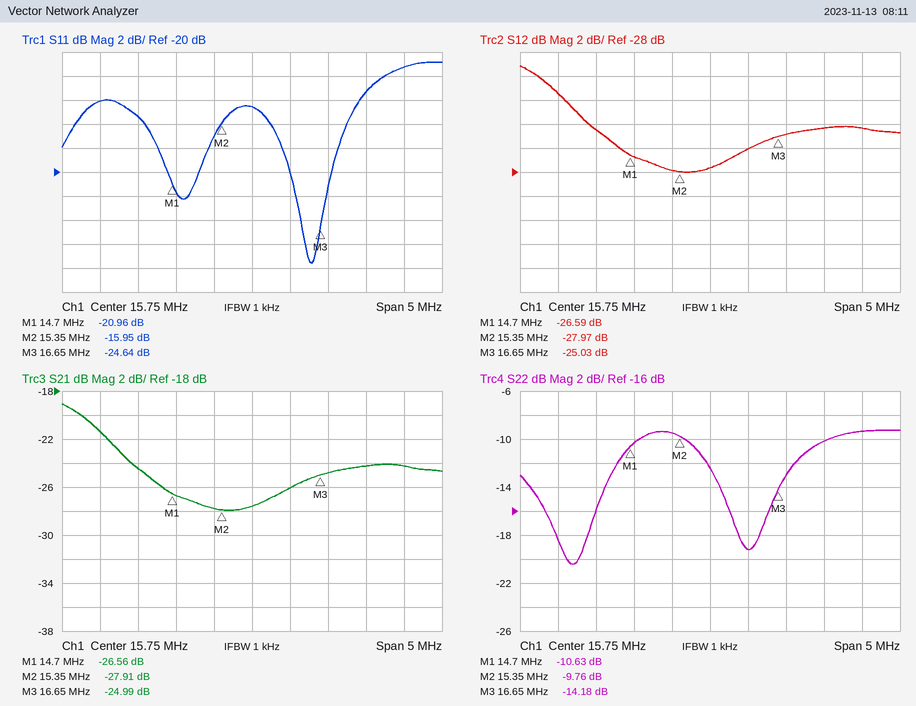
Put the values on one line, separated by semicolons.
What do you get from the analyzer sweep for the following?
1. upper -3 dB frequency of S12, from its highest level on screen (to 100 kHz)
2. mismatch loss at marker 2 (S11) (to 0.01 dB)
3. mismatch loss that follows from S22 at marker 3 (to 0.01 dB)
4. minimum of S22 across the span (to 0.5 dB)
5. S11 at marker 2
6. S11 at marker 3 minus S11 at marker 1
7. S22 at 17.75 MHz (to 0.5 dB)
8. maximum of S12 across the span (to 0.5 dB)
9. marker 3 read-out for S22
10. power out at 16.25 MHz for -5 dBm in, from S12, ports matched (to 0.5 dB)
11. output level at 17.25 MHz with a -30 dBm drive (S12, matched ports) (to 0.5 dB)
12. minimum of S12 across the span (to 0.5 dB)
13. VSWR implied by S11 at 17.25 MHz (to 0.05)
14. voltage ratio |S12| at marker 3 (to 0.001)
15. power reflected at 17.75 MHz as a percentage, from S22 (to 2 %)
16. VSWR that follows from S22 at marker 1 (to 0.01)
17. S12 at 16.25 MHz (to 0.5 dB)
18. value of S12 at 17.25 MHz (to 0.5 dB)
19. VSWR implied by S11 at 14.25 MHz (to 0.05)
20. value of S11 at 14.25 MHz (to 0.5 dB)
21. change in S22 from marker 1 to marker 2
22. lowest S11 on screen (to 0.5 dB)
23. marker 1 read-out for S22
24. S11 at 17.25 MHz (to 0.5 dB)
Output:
13.9 MHz; 0.11 dB; 0.17 dB; -20.5 dB; -15.95 dB; -3.68 dB; -9.5 dB; -19.0 dB; -14.18 dB; -31.0 dBm; -54.5 dBm; -28.0 dB; 1.55; 0.056; 12 %; 1.83; -26.0 dB; -24.5 dB; 1.40; -15.5 dB; 0.87 dB; -27.5 dB; -10.63 dB; -13.5 dB
